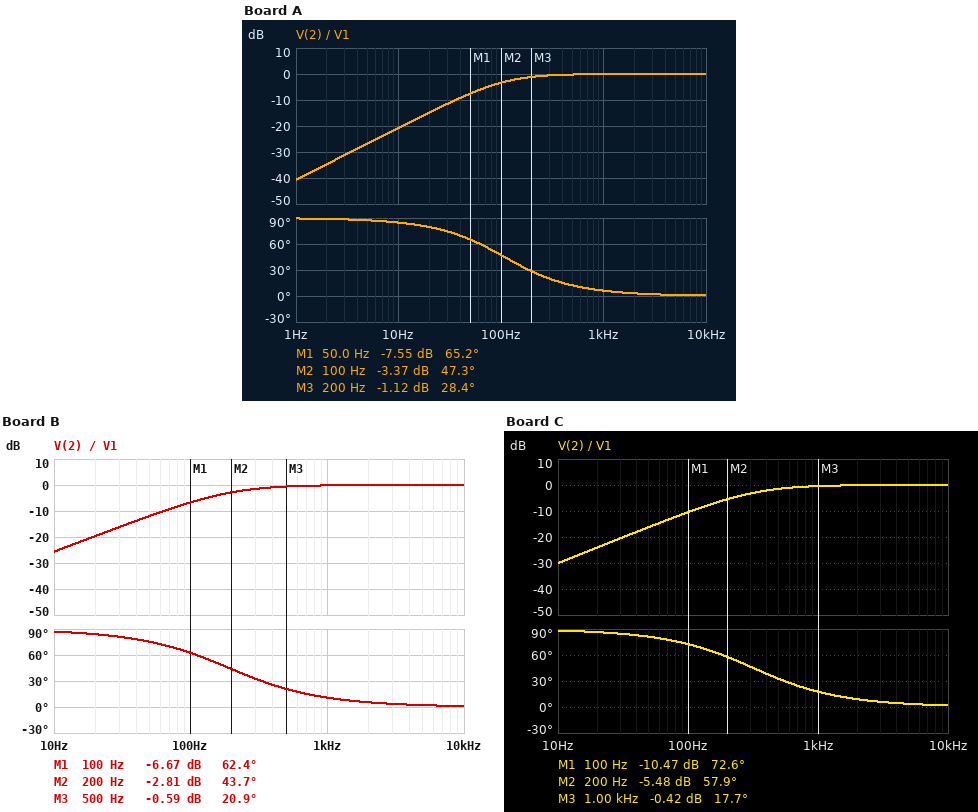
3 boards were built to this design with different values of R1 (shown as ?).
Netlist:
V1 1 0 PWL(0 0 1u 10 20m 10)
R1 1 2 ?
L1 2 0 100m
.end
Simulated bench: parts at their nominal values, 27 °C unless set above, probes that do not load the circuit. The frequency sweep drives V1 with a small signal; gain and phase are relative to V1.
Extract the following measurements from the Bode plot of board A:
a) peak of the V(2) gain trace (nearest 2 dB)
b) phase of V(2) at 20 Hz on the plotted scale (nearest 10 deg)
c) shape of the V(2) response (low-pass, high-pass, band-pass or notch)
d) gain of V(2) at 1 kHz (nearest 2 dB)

0 dB
80 deg
high-pass
0 dB
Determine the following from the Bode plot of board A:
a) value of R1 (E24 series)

68 Ω
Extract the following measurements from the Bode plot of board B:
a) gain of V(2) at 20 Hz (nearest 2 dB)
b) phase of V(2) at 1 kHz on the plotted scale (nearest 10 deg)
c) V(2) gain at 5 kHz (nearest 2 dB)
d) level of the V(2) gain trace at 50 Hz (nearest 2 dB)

-20 dB
10 deg
0 dB
-12 dB
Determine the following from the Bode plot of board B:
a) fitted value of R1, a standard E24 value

120 Ω
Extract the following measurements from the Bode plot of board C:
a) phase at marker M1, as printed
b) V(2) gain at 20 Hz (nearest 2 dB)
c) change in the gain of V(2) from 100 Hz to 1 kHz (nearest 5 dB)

72.6 deg
-24 dB
10 dB
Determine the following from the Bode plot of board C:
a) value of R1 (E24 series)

200 Ω
